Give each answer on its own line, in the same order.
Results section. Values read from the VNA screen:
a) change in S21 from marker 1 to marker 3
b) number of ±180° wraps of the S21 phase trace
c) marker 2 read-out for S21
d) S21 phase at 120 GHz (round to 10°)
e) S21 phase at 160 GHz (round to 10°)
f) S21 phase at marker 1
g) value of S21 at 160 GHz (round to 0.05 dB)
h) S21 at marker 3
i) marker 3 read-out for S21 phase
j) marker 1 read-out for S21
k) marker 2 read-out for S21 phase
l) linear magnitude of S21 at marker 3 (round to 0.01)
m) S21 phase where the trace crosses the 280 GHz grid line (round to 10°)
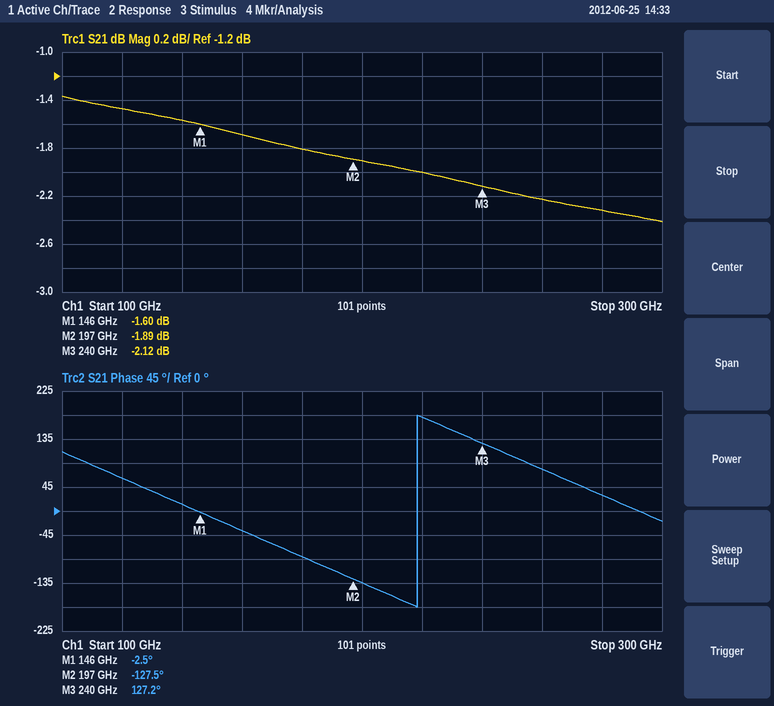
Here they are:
-0.52 dB
1
-1.89 dB
60°
-40°
-2.5°
-1.70 dB
-2.12 dB
127.2°
-1.60 dB
-127.5°
0.78
30°
